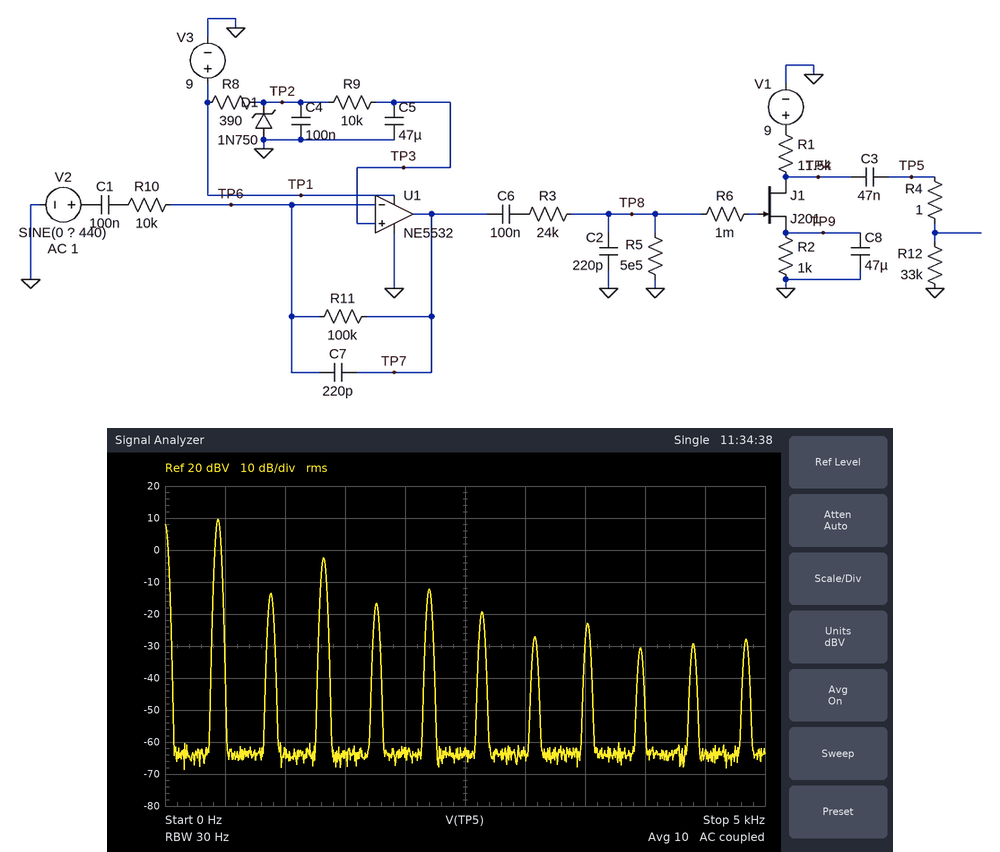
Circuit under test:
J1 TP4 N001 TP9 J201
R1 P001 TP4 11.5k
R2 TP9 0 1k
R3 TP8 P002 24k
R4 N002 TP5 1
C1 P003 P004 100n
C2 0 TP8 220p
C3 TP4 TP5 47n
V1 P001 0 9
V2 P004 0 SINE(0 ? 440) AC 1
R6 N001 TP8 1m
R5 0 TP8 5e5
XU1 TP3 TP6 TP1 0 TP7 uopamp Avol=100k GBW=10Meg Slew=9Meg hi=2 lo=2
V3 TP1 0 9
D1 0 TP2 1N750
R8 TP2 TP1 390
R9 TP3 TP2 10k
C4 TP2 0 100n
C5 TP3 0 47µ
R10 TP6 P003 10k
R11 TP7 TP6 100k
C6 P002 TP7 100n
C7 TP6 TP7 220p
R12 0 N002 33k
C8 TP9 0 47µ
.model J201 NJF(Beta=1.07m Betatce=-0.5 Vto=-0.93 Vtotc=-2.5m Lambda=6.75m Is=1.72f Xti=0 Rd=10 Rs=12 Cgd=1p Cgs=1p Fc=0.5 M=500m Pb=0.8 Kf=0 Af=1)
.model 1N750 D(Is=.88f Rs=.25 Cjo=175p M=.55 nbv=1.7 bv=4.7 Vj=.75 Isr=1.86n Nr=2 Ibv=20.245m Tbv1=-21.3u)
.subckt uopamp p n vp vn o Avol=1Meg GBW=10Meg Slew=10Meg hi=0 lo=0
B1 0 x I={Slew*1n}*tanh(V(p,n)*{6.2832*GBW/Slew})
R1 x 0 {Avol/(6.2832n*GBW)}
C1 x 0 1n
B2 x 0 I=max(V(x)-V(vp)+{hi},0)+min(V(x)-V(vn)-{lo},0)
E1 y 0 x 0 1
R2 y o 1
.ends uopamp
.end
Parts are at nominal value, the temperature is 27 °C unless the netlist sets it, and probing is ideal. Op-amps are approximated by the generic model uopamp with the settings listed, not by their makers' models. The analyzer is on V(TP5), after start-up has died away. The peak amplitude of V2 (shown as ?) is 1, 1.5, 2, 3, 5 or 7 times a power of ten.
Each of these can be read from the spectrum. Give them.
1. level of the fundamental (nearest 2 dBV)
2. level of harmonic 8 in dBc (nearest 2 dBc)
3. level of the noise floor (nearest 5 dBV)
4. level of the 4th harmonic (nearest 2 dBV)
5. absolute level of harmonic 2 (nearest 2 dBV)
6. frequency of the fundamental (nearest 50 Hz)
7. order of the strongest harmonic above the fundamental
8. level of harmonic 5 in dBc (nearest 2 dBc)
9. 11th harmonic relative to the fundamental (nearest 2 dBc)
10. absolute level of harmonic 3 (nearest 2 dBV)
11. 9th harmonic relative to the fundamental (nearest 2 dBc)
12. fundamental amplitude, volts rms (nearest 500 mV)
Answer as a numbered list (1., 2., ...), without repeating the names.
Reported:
1. 10 dBV
2. -32 dBc
3. -65 dBV
4. -16 dBV
5. -14 dBV
6. 450 Hz
7. 3
8. -22 dBc
9. -38 dBc
10. -2 dBV
11. -40 dBc
12. 3.0 V
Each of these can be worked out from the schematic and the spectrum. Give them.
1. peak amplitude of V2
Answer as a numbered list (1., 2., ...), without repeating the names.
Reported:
1. 100 mV
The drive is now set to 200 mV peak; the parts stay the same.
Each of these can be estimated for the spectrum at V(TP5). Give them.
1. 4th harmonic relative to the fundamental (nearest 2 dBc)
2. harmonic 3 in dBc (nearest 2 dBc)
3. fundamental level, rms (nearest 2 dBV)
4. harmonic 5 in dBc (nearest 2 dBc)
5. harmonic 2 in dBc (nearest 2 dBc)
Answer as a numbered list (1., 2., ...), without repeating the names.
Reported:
1. -12 dBc
2. -16 dBc
3. 10 dBV
4. -28 dBc
5. -10 dBc
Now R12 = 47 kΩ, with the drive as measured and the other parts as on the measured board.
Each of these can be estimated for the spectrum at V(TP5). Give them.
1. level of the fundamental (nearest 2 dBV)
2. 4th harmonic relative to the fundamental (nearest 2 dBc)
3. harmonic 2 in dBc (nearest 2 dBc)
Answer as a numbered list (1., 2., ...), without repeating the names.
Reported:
1. 10 dBV
2. -28 dBc
3. -26 dBc
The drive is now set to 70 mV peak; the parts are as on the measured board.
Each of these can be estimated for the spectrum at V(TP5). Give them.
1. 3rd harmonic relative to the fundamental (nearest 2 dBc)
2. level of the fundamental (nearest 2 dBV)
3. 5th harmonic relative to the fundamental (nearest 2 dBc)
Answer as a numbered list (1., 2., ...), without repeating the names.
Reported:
1. -14 dBc
2. 10 dBV
3. -34 dBc
